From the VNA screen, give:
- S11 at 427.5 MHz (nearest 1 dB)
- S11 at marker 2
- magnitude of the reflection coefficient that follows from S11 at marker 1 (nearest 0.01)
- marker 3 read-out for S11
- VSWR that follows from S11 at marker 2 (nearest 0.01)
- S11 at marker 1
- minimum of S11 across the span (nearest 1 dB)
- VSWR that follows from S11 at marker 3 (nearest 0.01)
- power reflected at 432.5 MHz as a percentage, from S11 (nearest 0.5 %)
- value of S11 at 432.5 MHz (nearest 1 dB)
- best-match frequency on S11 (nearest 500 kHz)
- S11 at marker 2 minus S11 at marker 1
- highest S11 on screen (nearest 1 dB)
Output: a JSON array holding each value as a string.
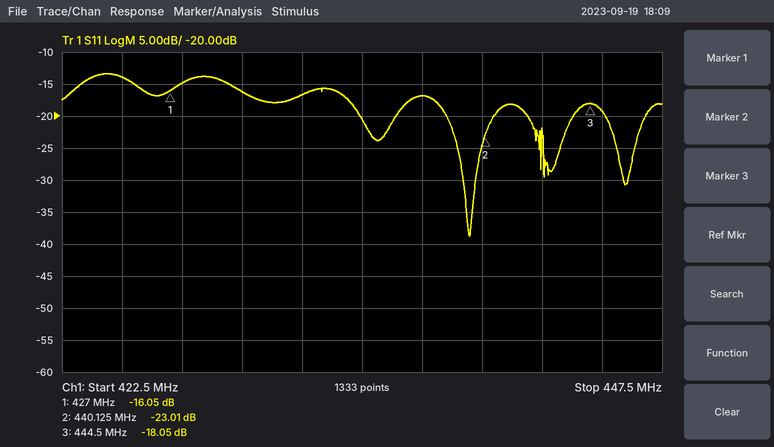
["-15 dB", "-23.01 dB", "0.16", "-18.05 dB", "1.15", "-16.05 dB", "-39 dB", "1.29", "2.0 %", "-17 dB", "439.5 MHz", "-6.96 dB", "-13 dB"]
